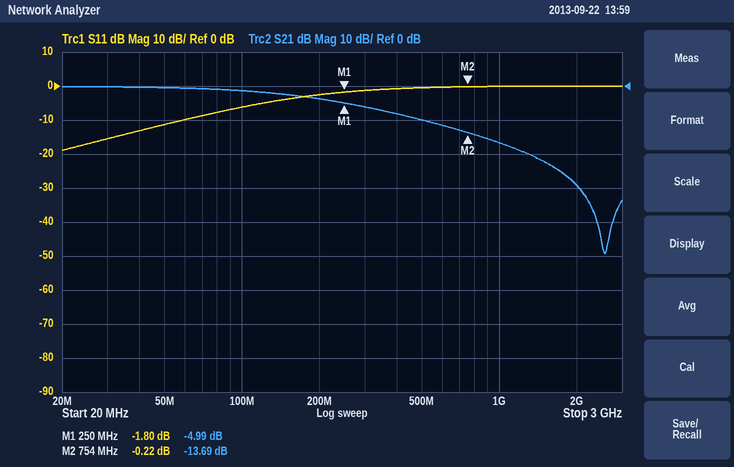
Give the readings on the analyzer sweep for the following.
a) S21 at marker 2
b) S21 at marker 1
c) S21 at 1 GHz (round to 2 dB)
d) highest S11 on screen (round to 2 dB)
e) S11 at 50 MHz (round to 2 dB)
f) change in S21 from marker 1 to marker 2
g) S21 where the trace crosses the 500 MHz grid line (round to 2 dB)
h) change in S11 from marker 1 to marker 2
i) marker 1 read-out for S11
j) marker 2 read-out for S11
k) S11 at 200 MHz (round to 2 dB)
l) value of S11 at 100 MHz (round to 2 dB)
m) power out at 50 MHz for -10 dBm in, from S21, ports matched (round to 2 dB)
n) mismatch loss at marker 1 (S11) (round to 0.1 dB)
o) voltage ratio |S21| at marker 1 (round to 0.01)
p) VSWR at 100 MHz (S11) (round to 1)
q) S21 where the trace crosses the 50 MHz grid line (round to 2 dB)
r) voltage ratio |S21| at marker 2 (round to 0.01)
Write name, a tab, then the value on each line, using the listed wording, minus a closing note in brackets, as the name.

S21 at marker 2	-13.69 dB
S21 at marker 1	-4.99 dB
S21 at 1 GHz	-16 dB
highest S11 on screen	0 dB
S11 at 50 MHz	-12 dB
change in S21 from marker 1 to marker 2	-8.70 dB
S21 where the trace crosses the 500 MHz grid line	-10 dB
change in S11 from marker 1 to marker 2	1.58 dB
marker 1 read-out for S11	-1.80 dB
marker 2 read-out for S11	-0.22 dB
S11 at 200 MHz	-2 dB
value of S11 at 100 MHz	-6 dB
power out at 50 MHz for -10 dBm in, from S21, ports matched	-10 dBm
mismatch loss at marker 1 (S11)	4.7 dB
voltage ratio |S21| at marker 1	0.56
VSWR at 100 MHz (S11)	3
S21 where the trace crosses the 50 MHz grid line	0 dB
voltage ratio |S21| at marker 2	0.21
